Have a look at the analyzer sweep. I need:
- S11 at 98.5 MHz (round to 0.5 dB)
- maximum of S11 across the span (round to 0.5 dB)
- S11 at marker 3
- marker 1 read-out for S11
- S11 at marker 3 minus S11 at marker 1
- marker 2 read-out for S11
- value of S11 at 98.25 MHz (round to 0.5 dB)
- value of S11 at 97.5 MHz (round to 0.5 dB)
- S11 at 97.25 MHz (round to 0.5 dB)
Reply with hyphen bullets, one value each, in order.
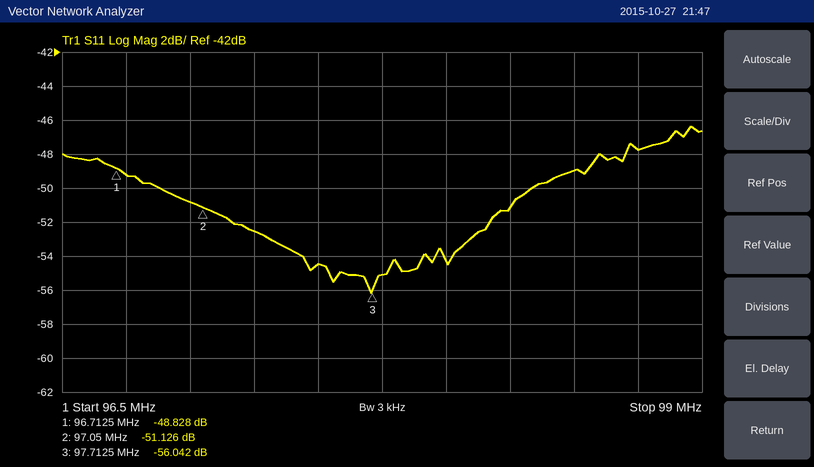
- -49.0 dB
- -46.5 dB
- -56.042 dB
- -48.828 dB
- -7.214 dB
- -51.126 dB
- -51.0 dB
- -54.5 dB
- -52.5 dB
